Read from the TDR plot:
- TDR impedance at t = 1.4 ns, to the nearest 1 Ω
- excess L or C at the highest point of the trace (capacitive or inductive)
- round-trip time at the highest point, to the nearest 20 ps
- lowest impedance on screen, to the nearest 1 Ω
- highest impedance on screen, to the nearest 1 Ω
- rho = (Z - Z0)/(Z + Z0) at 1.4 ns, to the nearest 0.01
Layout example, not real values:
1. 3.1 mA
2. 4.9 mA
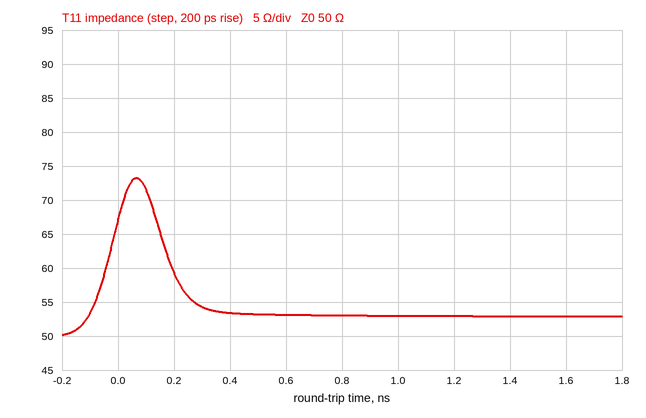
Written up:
1. 53 Ω
2. inductive
3. 60 ps
4. 50 Ω
5. 73 Ω
6. +0.03
